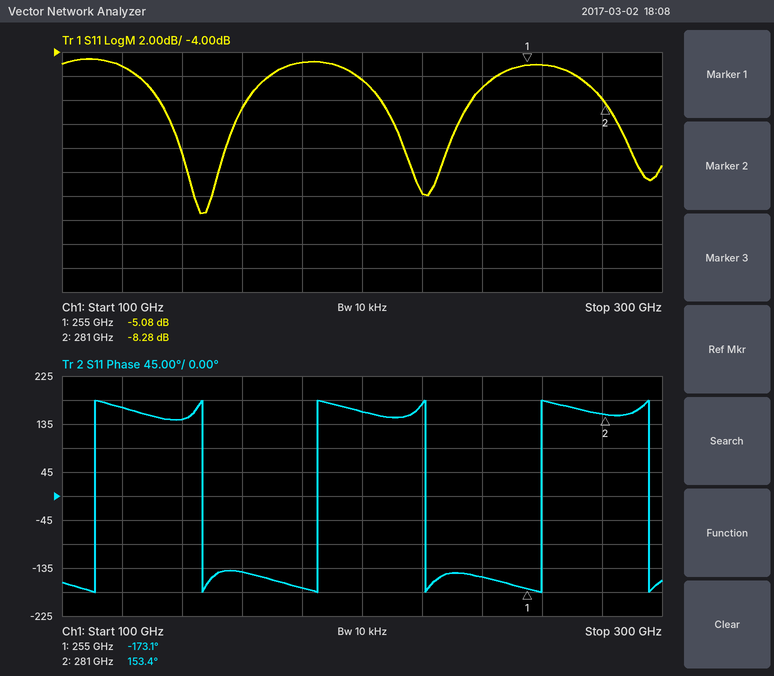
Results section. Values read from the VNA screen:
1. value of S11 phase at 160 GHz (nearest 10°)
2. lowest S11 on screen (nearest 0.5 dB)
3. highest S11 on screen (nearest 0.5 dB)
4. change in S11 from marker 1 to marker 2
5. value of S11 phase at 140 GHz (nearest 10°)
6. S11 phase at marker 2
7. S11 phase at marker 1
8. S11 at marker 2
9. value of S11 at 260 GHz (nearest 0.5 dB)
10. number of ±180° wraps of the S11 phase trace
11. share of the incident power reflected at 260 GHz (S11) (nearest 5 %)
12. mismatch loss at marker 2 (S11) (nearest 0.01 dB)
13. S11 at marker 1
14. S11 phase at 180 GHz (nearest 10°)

-140°
-17.5 dB
-4.5 dB
-3.20 dB
140°
153.4°
-173.1°
-8.28 dB
-5.0 dB
6
30 %
0.70 dB
-5.08 dB
-170°
